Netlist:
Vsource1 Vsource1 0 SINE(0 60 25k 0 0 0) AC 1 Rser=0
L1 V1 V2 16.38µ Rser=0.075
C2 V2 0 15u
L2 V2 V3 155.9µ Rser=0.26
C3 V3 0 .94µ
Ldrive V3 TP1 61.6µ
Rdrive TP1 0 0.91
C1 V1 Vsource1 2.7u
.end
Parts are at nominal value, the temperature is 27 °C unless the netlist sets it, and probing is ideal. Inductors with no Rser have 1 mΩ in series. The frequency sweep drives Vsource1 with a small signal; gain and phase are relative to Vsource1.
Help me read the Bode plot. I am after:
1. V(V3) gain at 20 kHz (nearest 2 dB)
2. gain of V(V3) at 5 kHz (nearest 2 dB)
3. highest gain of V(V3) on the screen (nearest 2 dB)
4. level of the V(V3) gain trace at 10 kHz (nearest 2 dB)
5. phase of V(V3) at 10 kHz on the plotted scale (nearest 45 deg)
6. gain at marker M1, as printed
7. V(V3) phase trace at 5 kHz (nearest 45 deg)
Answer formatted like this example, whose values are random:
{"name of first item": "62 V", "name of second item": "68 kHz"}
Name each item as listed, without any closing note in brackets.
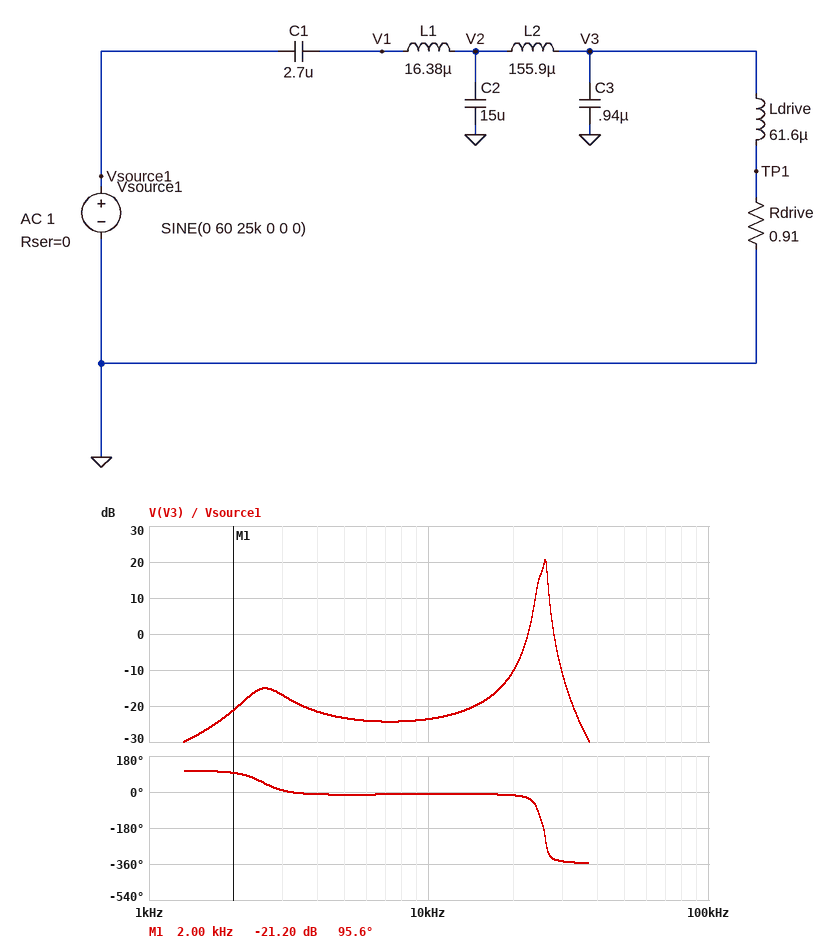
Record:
{"V(V3) gain at 20 kHz": "-10 dB", "gain of V(V3) at 5 kHz": "-24 dB", "highest gain of V(V3) on the screen": "20 dB", "level of the V(V3) gain trace at 10 kHz": "-24 dB", "phase of V(V3) at 10 kHz on the plotted scale": "0 deg", "gain at marker M1, as printed": "-21.20 dB", "V(V3) phase trace at 5 kHz": "0 deg"}
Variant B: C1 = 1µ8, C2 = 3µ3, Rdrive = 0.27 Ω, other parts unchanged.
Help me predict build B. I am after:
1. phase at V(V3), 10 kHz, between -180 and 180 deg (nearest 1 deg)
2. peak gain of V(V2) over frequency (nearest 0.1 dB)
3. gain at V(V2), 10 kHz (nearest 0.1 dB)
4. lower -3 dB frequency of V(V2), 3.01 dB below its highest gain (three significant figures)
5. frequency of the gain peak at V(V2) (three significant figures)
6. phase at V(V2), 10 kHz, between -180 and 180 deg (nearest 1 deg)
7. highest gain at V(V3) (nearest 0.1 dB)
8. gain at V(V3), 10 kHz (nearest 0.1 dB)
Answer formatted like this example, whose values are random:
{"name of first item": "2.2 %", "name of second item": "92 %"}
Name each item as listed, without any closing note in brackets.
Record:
{"phase at V(V3), 10 kHz, between -180 and 180 deg": "-2 deg", "peak gain of V(V2) over frequency": "25.2 dB", "gain at V(V2), 10 kHz": "-6.4 dB", "lower -3 dB frequency of V(V2), 3.01 dB below its highest gain": "36.4 kHz", "frequency of the gain peak at V(V2)": "36.7 kHz", "phase at V(V2), 10 kHz, between -180 and 180 deg": "0 deg", "highest gain at V(V3)": "18.1 dB", "gain at V(V3), 10 kHz": "-15.8 dB"}
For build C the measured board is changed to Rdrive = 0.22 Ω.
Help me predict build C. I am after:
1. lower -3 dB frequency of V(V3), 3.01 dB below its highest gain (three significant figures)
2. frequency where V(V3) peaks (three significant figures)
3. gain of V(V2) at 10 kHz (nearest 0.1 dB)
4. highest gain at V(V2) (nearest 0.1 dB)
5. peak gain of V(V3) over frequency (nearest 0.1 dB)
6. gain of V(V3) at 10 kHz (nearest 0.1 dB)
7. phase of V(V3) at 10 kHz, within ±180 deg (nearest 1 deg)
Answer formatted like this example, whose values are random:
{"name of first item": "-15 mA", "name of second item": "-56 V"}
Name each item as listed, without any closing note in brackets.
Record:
{"lower -3 dB frequency of V(V3), 3.01 dB below its highest gain": "24.5 kHz", "frequency where V(V3) peaks": "24.7 kHz", "gain of V(V2) at 10 kHz": "-14.4 dB", "highest gain at V(V2)": "14.8 dB", "peak gain of V(V3) over frequency": "25.9 dB", "gain of V(V3) at 10 kHz": "-23.8 dB", "phase of V(V3) at 10 kHz, within ±180 deg": "-2 deg"}
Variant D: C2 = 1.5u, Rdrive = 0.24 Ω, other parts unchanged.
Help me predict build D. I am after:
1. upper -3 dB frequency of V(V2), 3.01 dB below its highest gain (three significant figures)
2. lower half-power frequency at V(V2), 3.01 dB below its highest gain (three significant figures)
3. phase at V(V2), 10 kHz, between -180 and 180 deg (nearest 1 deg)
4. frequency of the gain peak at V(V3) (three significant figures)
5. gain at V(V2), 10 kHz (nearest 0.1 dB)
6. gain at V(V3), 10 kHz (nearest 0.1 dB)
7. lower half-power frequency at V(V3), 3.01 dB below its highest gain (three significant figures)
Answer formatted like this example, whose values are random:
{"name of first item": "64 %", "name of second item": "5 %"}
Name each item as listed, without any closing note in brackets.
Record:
{"upper -3 dB frequency of V(V2), 3.01 dB below its highest gain": "41.4 kHz", "lower half-power frequency at V(V2), 3.01 dB below its highest gain": "40.7 kHz", "phase at V(V2), 10 kHz, between -180 and 180 deg": "1 deg", "frequency of the gain peak at V(V3)": "24.7 kHz", "gain at V(V2), 10 kHz": "-1.1 dB", "gain at V(V3), 10 kHz": "-10.5 dB", "lower half-power frequency at V(V3), 3.01 dB below its highest gain": "24.4 kHz"}
